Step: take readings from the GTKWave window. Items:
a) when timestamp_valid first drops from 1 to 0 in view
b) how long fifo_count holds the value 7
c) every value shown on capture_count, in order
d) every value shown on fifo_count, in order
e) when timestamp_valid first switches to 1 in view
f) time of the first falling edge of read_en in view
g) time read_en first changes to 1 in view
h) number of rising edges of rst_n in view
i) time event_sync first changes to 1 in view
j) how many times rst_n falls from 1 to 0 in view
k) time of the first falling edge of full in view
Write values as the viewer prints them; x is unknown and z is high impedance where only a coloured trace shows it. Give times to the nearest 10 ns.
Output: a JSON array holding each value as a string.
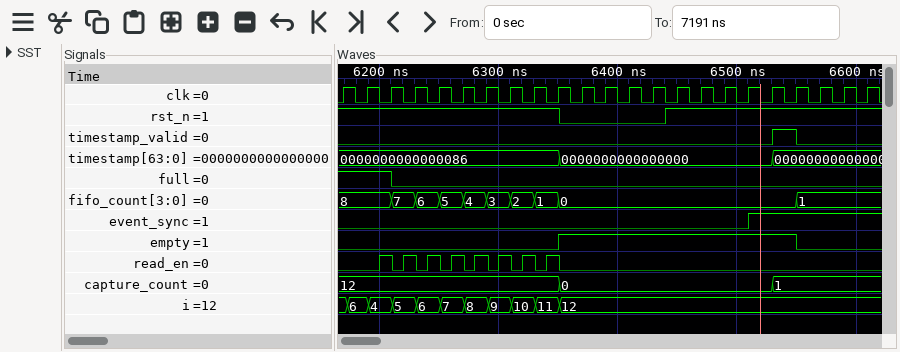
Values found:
["6550 ns", "20 ns", "12, 0, 1", "8, 7, 6, 5, 4, 3, 2, 1, 0, 1", "6530 ns", "6210 ns", "6200 ns", "1", "6510 ns", "1", "6210 ns"]
